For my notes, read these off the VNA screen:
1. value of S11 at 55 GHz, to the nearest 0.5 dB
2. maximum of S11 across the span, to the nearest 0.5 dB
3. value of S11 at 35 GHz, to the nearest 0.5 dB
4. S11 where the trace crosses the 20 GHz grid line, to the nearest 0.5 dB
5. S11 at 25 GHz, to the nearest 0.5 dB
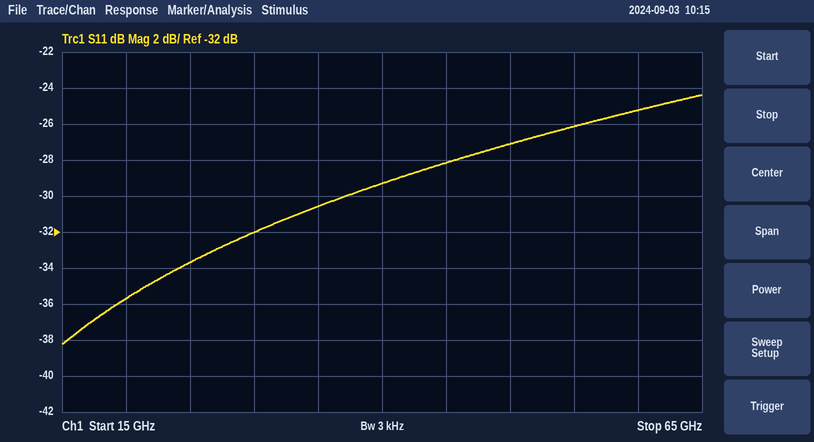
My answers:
-26.0 dB
-24.5 dB
-30.5 dB
-35.5 dB
-33.5 dB
